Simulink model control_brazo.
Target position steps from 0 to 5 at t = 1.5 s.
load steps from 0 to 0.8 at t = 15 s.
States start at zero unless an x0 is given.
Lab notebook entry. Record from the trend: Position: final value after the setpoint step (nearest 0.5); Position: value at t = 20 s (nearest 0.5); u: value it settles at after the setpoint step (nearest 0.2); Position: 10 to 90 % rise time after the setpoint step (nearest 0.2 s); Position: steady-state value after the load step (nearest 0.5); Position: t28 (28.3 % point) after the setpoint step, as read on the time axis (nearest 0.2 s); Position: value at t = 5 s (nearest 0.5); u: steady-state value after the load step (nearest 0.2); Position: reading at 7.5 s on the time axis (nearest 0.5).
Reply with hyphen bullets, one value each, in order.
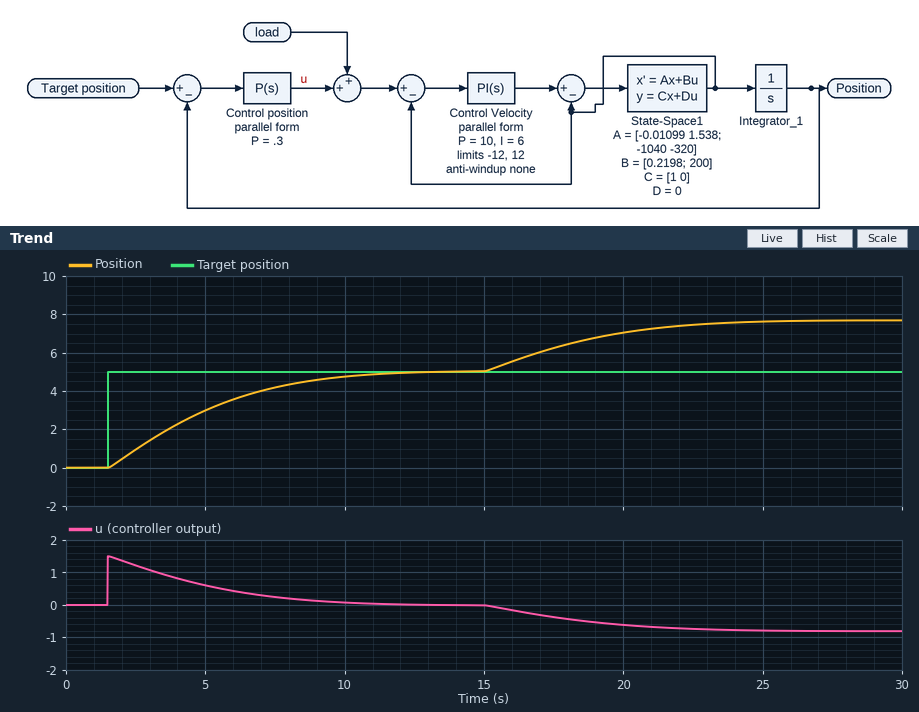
- 5.0
- 7.0
- 0.0
- 6.6 s
- 7.5
- 3.0 s
- 3.0
- -0.8
- 4.0
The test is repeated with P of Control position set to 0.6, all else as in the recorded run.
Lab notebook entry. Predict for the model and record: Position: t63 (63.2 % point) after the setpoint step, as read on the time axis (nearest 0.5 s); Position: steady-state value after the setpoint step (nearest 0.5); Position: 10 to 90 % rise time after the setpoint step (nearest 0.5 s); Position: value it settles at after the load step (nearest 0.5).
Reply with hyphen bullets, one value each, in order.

- 3.5 s
- 5.0
- 3.5 s
- 6.5
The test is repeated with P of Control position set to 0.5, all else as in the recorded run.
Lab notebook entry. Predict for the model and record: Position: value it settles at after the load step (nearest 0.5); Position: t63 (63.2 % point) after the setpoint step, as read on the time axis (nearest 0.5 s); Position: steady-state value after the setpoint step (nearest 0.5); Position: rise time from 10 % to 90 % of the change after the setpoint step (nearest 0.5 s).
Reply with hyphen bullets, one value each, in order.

- 6.5
- 4.0 s
- 5.0
- 4.0 s
